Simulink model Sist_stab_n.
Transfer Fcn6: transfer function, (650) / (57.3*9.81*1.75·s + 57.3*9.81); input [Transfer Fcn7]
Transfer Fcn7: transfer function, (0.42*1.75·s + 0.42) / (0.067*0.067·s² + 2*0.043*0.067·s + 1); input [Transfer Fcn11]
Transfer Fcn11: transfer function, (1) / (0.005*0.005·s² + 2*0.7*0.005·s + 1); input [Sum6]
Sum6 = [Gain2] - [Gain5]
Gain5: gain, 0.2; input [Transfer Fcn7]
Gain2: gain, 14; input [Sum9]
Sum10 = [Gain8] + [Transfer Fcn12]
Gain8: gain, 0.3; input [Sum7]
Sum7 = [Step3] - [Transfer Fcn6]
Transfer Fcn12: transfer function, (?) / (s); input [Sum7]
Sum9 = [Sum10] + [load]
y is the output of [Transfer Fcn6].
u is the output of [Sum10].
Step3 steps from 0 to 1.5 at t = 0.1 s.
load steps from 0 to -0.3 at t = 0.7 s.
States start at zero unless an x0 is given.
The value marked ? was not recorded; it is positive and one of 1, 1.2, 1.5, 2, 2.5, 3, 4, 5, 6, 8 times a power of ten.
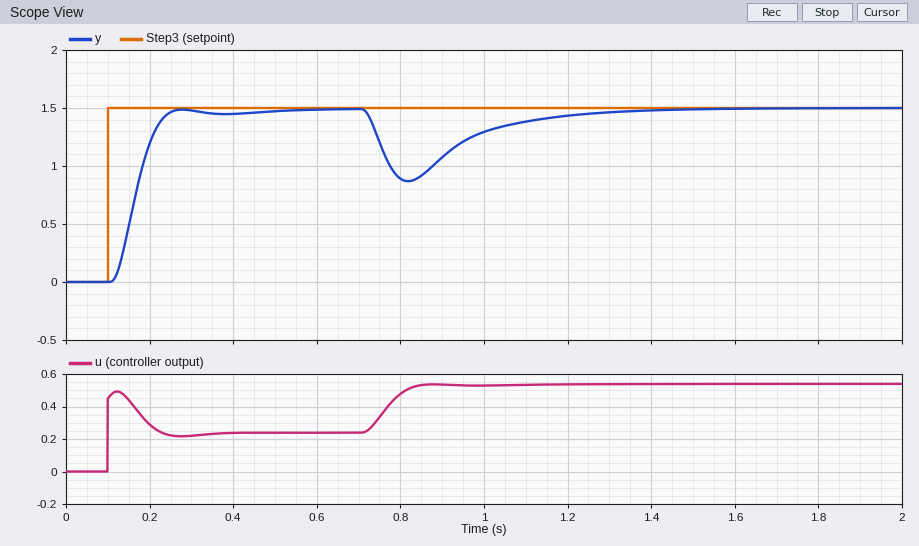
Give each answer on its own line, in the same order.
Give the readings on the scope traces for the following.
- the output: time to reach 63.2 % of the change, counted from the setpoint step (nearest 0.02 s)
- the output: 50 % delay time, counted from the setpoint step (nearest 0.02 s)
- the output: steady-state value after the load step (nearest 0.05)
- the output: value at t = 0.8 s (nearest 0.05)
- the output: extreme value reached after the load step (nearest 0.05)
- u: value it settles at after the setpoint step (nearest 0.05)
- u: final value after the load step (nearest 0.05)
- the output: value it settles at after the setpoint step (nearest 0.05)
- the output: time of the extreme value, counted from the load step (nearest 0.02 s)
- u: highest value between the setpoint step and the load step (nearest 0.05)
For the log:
0.08 s
0.06 s
1.50
0.90
0.85
0.25
0.55
1.50
0.12 s
0.50
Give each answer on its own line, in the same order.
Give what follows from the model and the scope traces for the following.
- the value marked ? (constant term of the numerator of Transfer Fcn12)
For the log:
2
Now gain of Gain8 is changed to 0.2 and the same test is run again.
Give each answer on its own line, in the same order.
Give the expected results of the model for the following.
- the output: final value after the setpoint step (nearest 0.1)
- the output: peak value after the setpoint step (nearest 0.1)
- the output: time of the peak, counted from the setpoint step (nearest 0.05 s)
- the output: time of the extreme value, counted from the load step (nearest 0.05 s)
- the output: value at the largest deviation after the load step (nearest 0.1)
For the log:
1.5
1.6
0.25 s
0.15 s
0.8
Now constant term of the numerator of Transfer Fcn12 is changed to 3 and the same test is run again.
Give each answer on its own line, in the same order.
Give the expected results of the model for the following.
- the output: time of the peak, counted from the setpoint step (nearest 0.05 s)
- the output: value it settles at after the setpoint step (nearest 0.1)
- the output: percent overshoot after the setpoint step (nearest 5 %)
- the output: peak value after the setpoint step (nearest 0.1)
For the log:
0.15 s
1.5
10 %
1.7
